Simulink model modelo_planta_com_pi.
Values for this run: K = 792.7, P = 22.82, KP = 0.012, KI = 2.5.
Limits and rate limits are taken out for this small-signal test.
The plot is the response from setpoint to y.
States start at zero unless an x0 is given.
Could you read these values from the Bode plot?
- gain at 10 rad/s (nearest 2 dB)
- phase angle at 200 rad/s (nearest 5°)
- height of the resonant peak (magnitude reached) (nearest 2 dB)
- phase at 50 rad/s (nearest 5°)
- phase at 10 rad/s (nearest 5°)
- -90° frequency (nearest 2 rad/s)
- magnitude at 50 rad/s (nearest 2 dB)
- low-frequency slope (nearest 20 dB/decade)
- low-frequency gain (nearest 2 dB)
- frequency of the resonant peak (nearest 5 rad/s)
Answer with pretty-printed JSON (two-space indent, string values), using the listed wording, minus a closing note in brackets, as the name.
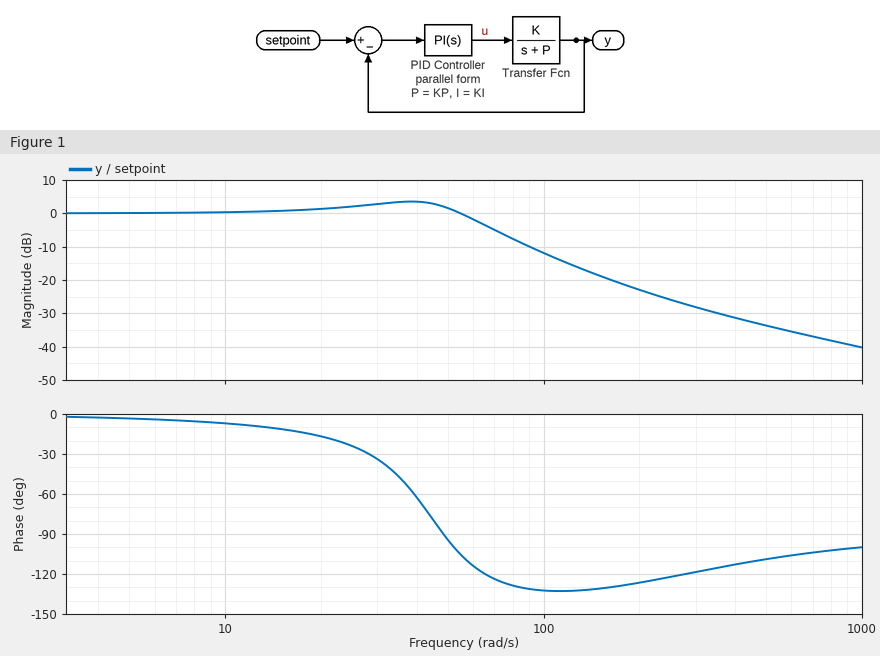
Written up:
{
  "gain at 10 rad/s": "0 dB",
  "phase angle at 200 rad/s": "-125°",
  "height of the resonant peak (magnitude reached)": "4 dB",
  "phase at 50 rad/s": "-95°",
  "phase at 10 rad/s": "-5°",
  "-90° frequency": "48 rad/s",
  "magnitude at 50 rad/s": "2 dB",
  "low-frequency slope": "0 dB/decade",
  "low-frequency gain": "0 dB",
  "frequency of the resonant peak": "40 rad/s"
}
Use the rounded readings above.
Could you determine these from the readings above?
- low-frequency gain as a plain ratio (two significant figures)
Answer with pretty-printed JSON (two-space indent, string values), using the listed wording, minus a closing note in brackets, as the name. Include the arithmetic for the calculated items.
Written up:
{
  "low-frequency gain as a plain ratio": "10^(0 / 20) = 1.0"
}
